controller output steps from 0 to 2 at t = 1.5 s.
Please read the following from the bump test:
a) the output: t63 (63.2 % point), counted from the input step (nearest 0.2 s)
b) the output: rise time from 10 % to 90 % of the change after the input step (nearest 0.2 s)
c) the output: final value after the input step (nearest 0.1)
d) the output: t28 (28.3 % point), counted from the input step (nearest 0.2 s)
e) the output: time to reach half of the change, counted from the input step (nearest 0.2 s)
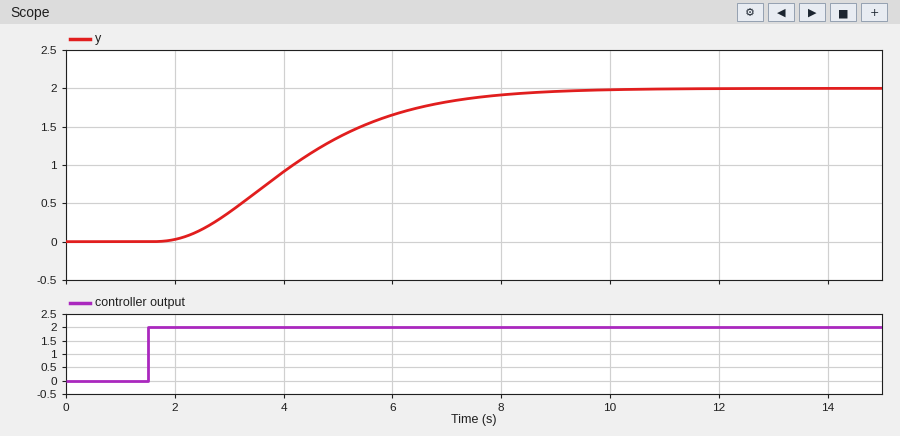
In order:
3.2 s
4.2 s
2.0
1.8 s
2.6 s
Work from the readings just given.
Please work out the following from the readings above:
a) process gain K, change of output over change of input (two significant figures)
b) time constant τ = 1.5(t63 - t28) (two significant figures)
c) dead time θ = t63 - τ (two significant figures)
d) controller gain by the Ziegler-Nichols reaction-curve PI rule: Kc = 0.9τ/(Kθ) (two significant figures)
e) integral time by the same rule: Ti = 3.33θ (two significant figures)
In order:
1.0
2.1 s
1.1 s
1.7
3.7 s
